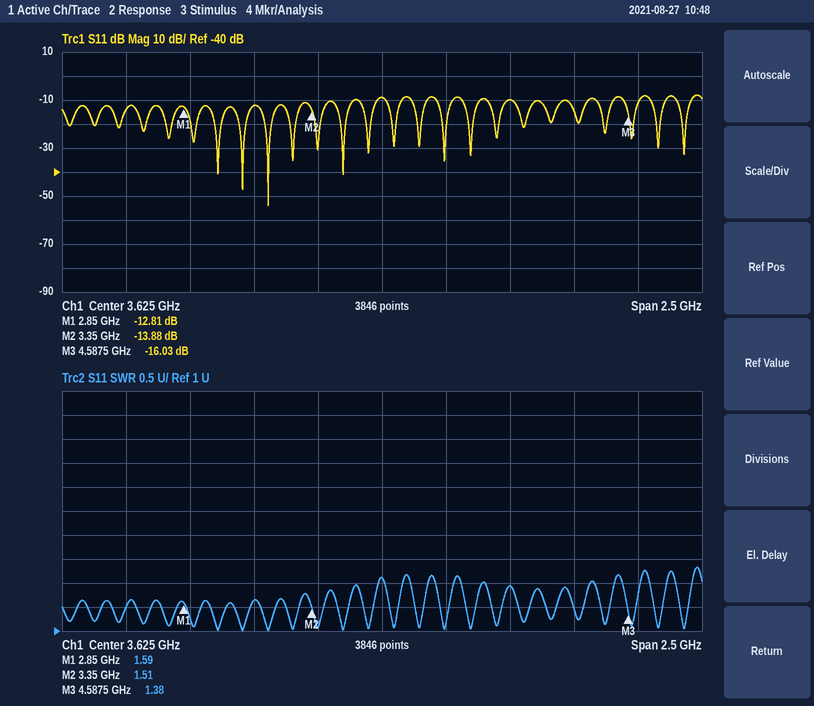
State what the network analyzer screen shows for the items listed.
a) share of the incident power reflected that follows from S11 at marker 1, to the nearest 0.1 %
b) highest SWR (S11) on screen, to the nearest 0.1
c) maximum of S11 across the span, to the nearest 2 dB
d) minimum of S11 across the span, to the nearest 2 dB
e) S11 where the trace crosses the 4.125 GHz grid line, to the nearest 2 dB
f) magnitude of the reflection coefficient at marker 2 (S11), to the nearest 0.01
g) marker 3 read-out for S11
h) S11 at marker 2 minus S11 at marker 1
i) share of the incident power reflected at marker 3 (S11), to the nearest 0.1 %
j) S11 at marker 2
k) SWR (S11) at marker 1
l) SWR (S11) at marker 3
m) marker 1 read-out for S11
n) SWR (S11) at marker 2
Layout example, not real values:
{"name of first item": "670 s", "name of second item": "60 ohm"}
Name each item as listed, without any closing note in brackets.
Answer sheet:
{"share of the incident power reflected that follows from S11 at marker 1, to the nearest 0.1 %": "5.2 %", "highest SWR (S11) on screen, to the nearest 0.1": "2.3", "maximum of S11 across the span, to the nearest 2 dB": "-8 dB", "minimum of S11 across the span, to the nearest 2 dB": "-54 dB", "S11 where the trace crosses the 4.125 GHz grid line, to the nearest 2 dB": "-10 dB", "magnitude of the reflection coefficient at marker 2 (S11), to the nearest 0.01": "0.20", "marker 3 read-out for S11": "-16.03 dB", "S11 at marker 2 minus S11 at marker 1": "-1.07 dB", "share of the incident power reflected at marker 3 (S11), to the nearest 0.1 %": "2.5 %", "S11 at marker 2": "-13.88 dB", "SWR (S11) at marker 1": "1.59", "SWR (S11) at marker 3": "1.38", "marker 1 read-out for S11": "-12.81 dB", "SWR (S11) at marker 2": "1.51"}
